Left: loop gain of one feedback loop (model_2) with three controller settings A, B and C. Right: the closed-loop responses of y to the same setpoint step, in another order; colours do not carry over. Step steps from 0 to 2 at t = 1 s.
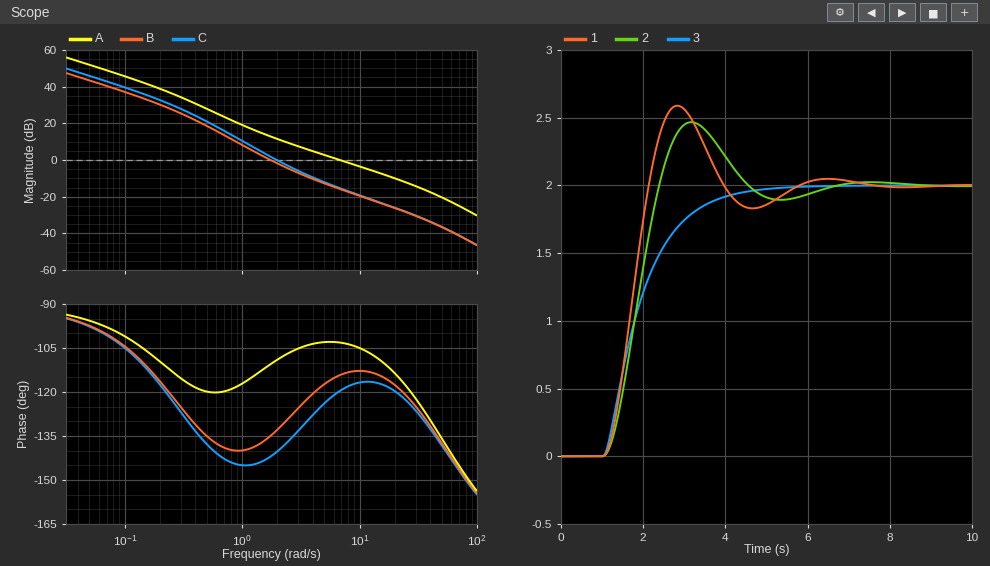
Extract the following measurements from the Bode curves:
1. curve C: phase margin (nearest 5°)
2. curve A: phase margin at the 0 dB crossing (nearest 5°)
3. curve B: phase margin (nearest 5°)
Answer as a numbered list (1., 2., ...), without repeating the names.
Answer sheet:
1. 40°
2. 75°
3. 45°
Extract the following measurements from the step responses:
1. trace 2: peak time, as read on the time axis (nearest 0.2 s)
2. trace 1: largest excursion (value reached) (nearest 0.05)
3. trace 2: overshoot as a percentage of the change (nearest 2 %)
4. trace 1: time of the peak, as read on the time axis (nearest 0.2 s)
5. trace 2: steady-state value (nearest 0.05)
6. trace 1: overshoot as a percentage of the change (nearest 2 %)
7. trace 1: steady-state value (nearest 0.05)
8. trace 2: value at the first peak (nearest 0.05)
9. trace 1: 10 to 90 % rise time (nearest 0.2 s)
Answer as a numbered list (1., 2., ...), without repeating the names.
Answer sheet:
1. 3.2 s
2. 2.60
3. 24 %
4. 2.8 s
5. 2.00
6. 30 %
7. 2.00
8. 2.45
9. 0.8 s
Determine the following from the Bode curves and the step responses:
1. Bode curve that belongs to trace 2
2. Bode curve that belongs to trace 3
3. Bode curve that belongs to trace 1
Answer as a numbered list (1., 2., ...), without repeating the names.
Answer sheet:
1. B
2. A
3. C
